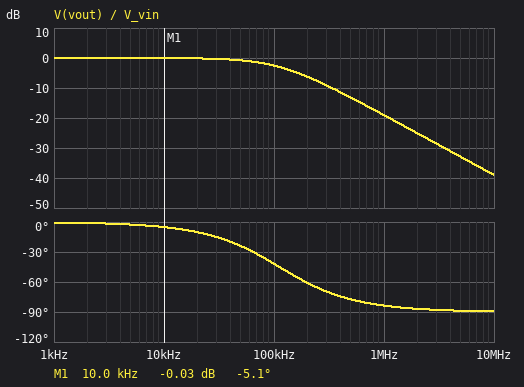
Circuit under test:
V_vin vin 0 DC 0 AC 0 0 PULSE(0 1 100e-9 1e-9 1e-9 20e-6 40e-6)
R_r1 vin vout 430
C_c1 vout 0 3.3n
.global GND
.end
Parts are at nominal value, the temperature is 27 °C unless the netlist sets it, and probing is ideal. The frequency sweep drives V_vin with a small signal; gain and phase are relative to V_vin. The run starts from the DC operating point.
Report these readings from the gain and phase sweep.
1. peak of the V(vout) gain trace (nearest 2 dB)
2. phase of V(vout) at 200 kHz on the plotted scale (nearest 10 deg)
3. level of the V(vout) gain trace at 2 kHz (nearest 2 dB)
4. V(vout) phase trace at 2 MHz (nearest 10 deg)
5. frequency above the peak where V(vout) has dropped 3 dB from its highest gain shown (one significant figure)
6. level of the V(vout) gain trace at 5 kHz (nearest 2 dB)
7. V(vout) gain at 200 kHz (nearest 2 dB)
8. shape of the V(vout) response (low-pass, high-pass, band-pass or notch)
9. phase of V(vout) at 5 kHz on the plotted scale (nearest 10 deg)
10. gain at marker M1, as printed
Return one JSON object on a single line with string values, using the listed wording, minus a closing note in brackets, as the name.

{"peak of the V(vout) gain trace": "0 dB", "phase of V(vout) at 200 kHz on the plotted scale": "-60 deg", "level of the V(vout) gain trace at 2 kHz": "0 dB", "V(vout) phase trace at 2 MHz": "-90 deg", "frequency above the peak where V(vout) has dropped 3 dB from its highest gain shown": "100 kHz", "level of the V(vout) gain trace at 5 kHz": "0 dB", "V(vout) gain at 200 kHz": "-6 dB", "shape of the V(vout) response": "low-pass", "phase of V(vout) at 5 kHz on the plotted scale": "0 deg", "gain at marker M1, as printed": "-0.03 dB"}
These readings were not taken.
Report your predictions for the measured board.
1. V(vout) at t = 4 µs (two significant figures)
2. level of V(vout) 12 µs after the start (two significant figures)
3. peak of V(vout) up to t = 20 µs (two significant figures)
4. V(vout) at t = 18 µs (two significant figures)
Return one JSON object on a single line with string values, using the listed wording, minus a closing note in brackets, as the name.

{"V(vout) at t = 4 µs": "940 mV", "level of V(vout) 12 µs after the start": "1.0 V", "peak of V(vout) up to t = 20 µs": "1.0 V", "V(vout) at t = 18 µs": "1.0 V"}
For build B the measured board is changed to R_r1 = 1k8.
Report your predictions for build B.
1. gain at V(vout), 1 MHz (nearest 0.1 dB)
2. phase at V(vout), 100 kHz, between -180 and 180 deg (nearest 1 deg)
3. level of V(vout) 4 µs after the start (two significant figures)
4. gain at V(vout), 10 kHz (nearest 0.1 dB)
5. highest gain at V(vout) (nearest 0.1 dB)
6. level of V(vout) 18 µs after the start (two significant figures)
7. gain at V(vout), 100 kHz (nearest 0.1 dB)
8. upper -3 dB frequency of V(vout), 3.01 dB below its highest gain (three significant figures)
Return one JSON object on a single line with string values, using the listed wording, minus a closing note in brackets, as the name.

{"gain at V(vout), 1 MHz": "-31.4 dB", "phase at V(vout), 100 kHz, between -180 and 180 deg": "-75 deg", "level of V(vout) 4 µs after the start": "480 mV", "gain at V(vout), 10 kHz": "-0.6 dB", "highest gain at V(vout)": "0 dB", "level of V(vout) 18 µs after the start": "950 mV", "gain at V(vout), 100 kHz": "-11.7 dB", "upper -3 dB frequency of V(vout), 3.01 dB below its highest gain": "26.8 kHz"}
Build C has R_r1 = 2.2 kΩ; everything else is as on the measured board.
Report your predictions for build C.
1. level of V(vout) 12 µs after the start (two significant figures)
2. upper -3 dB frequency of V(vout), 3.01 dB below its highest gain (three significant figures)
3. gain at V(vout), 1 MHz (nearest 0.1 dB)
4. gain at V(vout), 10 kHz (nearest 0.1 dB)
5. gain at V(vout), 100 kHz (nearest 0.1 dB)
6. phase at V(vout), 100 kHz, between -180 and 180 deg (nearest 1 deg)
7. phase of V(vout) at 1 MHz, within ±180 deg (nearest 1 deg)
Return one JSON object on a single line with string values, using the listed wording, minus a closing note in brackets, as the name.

{"level of V(vout) 12 µs after the start": "810 mV", "upper -3 dB frequency of V(vout), 3.01 dB below its highest gain": "21.9 kHz", "gain at V(vout), 1 MHz": "-33.2 dB", "gain at V(vout), 10 kHz": "-0.8 dB", "gain at V(vout), 100 kHz": "-13.4 dB", "phase at V(vout), 100 kHz, between -180 and 180 deg": "-78 deg", "phase of V(vout) at 1 MHz, within ±180 deg": "-89 deg"}
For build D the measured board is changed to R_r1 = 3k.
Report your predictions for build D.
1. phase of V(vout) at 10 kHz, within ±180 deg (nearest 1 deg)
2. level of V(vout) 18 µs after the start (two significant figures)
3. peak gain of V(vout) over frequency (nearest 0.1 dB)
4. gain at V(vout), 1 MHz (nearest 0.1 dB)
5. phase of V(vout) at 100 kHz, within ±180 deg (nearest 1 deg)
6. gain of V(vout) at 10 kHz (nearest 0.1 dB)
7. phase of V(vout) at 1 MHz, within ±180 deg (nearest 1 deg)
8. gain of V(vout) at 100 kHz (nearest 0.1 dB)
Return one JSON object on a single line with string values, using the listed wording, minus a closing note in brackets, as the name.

{"phase of V(vout) at 10 kHz, within ±180 deg": "-32 deg", "level of V(vout) 18 µs after the start": "840 mV", "peak gain of V(vout) over frequency": "0 dB", "gain at V(vout), 1 MHz": "-35.9 dB", "phase of V(vout) at 100 kHz, within ±180 deg": "-81 deg", "gain of V(vout) at 10 kHz": "-1.4 dB", "phase of V(vout) at 1 MHz, within ±180 deg": "-89 deg", "gain of V(vout) at 100 kHz": "-16.0 dB"}
